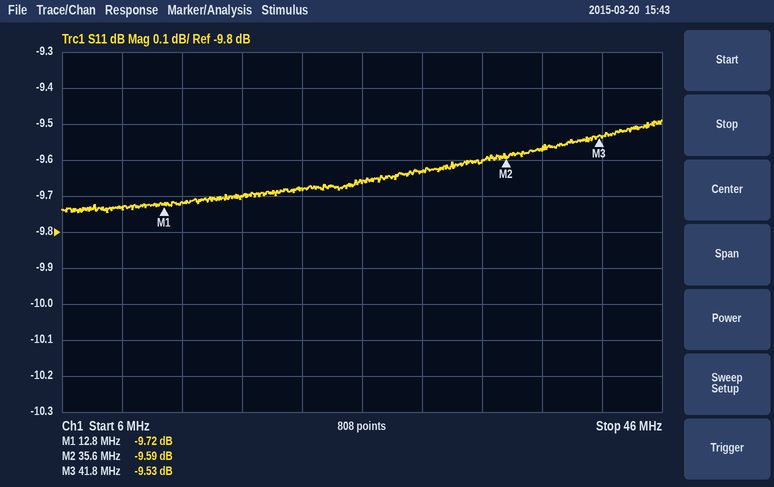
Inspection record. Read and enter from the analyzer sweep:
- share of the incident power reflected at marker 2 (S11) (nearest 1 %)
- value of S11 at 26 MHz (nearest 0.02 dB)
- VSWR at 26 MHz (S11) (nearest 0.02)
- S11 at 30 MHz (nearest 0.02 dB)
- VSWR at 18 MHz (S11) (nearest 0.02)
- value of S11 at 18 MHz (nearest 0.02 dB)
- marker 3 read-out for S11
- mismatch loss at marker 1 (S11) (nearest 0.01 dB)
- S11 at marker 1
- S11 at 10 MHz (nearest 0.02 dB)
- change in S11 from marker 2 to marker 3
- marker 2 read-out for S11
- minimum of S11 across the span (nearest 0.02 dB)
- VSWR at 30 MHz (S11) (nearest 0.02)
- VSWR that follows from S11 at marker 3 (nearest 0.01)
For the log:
11 %
-9.66 dB
1.98
-9.64 dB
1.98
-9.70 dB
-9.53 dB
0.49 dB
-9.72 dB
-9.74 dB
0.06 dB
-9.59 dB
-9.74 dB
1.98
2.00
